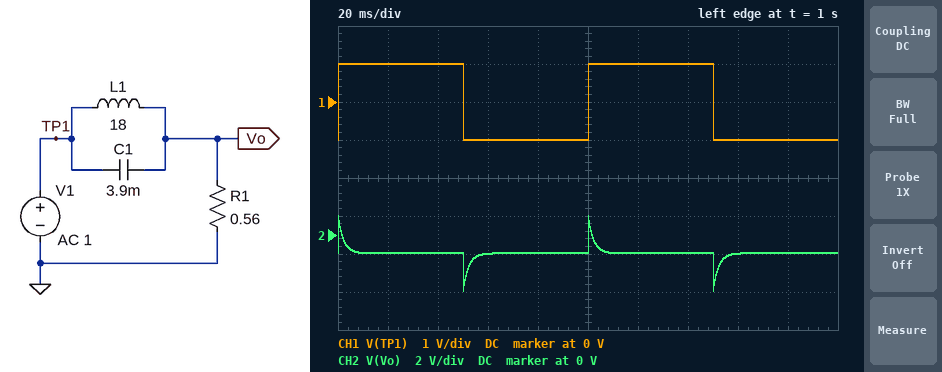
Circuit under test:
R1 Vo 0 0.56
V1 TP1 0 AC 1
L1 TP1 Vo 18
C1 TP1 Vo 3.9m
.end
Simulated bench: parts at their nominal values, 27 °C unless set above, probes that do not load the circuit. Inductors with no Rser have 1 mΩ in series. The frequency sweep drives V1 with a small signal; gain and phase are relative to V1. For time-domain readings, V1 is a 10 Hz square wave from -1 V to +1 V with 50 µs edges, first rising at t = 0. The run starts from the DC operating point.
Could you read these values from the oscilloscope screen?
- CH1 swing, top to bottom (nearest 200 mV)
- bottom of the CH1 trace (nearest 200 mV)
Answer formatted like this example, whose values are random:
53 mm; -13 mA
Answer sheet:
2.0 V; -1.0 V
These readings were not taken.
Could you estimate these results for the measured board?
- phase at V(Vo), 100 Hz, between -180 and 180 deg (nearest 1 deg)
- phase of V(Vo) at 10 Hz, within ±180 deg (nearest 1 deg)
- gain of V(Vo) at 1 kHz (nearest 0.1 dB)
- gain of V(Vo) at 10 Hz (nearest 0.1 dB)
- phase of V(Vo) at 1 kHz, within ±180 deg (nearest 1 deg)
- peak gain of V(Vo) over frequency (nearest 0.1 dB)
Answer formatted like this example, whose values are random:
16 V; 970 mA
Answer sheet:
36 deg; 82 deg; 0 dB; -17.4 dB; 4 deg; 0 dB
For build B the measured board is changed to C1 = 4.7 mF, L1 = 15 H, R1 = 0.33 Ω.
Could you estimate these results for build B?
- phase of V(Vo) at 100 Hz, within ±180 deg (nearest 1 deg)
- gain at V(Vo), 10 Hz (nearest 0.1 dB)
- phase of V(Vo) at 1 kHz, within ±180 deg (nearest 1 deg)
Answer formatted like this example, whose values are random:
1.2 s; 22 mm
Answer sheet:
46 deg; -20.3 dB; 6 deg
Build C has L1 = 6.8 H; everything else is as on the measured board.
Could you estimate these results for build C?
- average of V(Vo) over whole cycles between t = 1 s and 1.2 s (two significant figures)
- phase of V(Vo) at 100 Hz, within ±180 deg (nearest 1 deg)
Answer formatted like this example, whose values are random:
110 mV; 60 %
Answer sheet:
-910 mV; 36 deg
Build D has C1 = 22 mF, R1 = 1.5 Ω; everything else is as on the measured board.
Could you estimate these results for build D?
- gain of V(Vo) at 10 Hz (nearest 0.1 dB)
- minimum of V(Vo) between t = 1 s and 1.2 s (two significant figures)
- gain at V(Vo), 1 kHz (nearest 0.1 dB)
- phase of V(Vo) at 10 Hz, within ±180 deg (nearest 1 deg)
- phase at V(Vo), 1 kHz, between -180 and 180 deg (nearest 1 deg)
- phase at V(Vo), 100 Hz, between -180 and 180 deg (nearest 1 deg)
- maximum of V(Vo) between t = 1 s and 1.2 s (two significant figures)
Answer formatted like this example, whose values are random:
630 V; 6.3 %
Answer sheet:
-0.9 dB; -2.6 V; 0 dB; 26 deg; 0 deg; 3 deg; 720 mV
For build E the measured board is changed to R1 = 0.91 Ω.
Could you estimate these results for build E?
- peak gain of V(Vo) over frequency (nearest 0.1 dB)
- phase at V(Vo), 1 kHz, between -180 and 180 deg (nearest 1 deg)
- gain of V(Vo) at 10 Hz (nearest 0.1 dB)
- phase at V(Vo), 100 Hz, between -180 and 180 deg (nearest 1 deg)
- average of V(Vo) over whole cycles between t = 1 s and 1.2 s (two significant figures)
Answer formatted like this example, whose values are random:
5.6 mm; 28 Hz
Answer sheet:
0 dB; 3 deg; -13.3 dB; 24 deg; -900 mV
